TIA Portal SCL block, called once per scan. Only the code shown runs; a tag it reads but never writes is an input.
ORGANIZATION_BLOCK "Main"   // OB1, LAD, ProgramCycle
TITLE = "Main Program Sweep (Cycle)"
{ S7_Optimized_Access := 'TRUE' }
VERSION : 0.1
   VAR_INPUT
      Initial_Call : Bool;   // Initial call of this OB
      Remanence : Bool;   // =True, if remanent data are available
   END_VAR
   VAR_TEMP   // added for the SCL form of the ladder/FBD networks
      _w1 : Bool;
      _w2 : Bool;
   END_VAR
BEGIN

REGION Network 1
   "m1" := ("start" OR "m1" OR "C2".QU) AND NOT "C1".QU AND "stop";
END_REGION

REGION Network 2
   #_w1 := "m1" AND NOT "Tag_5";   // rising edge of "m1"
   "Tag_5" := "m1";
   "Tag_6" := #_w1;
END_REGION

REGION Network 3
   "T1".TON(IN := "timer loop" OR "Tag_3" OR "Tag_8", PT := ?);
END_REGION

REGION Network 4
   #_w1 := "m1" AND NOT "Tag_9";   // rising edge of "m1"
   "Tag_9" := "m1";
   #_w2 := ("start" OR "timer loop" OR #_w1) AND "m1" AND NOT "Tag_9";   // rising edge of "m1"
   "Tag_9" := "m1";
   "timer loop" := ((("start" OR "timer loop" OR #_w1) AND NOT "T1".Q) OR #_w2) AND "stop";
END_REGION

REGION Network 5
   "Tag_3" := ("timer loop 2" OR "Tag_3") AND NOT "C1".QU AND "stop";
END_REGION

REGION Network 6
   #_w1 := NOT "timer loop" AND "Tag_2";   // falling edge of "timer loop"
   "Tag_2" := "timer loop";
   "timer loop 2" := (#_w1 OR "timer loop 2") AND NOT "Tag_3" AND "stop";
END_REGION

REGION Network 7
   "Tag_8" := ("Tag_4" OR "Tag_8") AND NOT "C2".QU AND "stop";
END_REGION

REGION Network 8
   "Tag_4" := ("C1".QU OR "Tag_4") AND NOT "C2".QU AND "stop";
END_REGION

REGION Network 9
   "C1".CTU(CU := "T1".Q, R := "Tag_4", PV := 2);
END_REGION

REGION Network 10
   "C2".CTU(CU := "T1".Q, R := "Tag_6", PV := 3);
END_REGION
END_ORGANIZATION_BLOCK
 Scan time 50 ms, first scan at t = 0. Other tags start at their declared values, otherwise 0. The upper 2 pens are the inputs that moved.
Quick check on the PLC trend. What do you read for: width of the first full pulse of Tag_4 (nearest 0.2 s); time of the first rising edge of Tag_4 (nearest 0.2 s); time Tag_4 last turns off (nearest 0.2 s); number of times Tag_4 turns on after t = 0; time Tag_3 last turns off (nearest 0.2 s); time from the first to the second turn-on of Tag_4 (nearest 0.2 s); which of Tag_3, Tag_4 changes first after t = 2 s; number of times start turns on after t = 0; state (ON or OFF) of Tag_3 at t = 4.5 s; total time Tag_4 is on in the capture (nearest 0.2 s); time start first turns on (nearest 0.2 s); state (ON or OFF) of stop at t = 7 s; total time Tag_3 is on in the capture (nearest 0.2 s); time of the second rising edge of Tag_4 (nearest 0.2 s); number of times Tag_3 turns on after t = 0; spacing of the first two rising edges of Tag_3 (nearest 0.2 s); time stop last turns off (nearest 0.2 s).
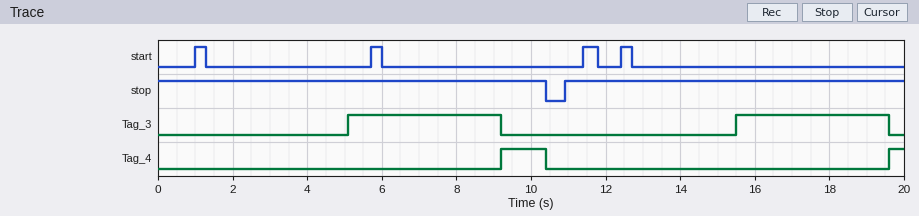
1.2 s
9.2 s
10.4 s
2
19.6 s
10.4 s
Tag_3
4
OFF
1.6 s
1.0 s
ON
8.2 s
19.6 s
2
10.4 s
10.4 s
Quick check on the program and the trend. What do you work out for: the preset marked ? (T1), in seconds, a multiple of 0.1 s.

4.0 s
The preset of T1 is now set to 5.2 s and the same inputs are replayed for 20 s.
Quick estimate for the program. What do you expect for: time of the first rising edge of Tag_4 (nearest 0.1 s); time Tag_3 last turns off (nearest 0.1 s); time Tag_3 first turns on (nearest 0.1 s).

16.7 s
10.4 s
6.3 s
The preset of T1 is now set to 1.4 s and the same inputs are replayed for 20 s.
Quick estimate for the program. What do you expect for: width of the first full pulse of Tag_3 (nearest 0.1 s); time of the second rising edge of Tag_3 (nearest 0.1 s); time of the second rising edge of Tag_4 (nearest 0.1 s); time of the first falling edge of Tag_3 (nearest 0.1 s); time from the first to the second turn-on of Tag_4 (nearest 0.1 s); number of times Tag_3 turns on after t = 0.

1.5 s
7.2 s
8.7 s
4.0 s
4.7 s
3
